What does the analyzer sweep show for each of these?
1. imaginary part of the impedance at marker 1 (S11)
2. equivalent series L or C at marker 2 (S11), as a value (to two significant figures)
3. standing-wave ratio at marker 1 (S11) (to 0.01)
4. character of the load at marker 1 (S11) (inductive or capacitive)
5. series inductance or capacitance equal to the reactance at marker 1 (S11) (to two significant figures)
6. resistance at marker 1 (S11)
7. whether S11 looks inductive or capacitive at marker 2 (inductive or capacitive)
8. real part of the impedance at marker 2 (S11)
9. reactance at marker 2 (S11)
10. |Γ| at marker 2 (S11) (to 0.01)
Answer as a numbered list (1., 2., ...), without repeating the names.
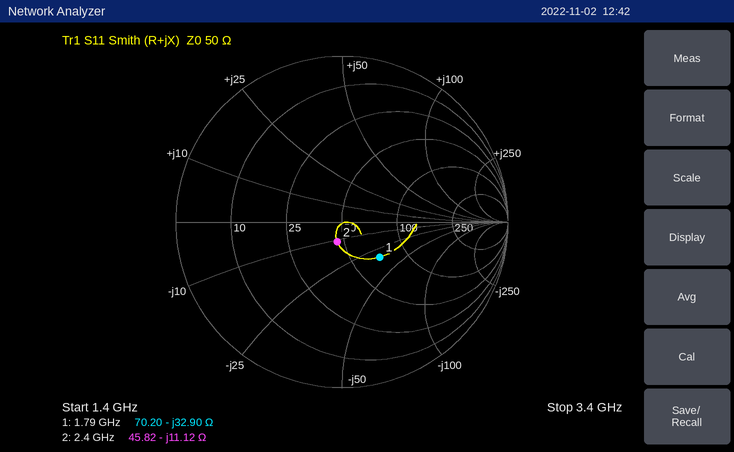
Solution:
1. -32.90 Ω
2. 6.0 pF
3. 1.90
4. capacitive
5. 2.7 pF
6. 70.20 Ω
7. capacitive
8. 45.82 Ω
9. -11.12 Ω
10. 0.12
